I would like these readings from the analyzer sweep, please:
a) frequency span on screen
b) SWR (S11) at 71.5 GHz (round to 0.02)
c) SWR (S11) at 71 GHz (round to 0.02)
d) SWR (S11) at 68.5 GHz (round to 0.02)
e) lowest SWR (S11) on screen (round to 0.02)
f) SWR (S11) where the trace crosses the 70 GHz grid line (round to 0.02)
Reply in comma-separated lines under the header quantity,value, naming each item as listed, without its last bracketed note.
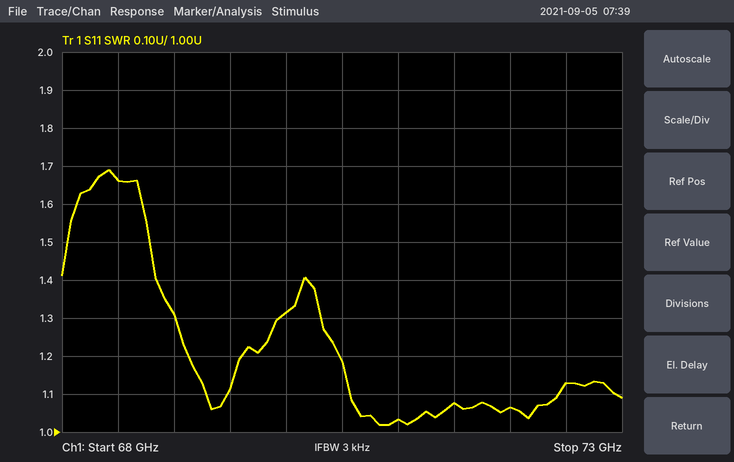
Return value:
quantity,value
frequency span on screen,5 GHz
SWR (S11) at 71.5 GHz,1.08
SWR (S11) at 71 GHz,1.04
SWR (S11) at 68.5 GHz,1.66
lowest SWR (S11) on screen,1.02
SWR (S11) where the trace crosses the 70 GHz grid line,1.32
